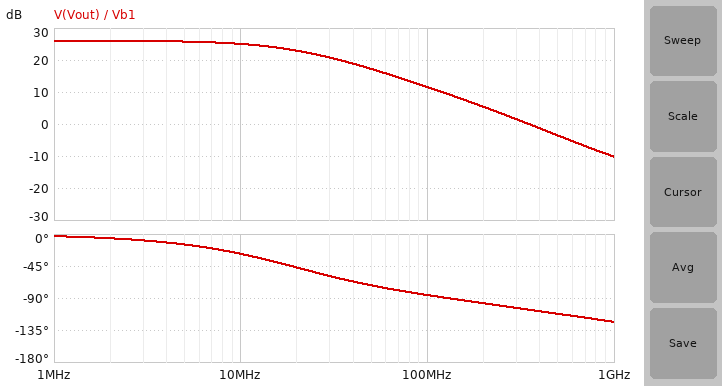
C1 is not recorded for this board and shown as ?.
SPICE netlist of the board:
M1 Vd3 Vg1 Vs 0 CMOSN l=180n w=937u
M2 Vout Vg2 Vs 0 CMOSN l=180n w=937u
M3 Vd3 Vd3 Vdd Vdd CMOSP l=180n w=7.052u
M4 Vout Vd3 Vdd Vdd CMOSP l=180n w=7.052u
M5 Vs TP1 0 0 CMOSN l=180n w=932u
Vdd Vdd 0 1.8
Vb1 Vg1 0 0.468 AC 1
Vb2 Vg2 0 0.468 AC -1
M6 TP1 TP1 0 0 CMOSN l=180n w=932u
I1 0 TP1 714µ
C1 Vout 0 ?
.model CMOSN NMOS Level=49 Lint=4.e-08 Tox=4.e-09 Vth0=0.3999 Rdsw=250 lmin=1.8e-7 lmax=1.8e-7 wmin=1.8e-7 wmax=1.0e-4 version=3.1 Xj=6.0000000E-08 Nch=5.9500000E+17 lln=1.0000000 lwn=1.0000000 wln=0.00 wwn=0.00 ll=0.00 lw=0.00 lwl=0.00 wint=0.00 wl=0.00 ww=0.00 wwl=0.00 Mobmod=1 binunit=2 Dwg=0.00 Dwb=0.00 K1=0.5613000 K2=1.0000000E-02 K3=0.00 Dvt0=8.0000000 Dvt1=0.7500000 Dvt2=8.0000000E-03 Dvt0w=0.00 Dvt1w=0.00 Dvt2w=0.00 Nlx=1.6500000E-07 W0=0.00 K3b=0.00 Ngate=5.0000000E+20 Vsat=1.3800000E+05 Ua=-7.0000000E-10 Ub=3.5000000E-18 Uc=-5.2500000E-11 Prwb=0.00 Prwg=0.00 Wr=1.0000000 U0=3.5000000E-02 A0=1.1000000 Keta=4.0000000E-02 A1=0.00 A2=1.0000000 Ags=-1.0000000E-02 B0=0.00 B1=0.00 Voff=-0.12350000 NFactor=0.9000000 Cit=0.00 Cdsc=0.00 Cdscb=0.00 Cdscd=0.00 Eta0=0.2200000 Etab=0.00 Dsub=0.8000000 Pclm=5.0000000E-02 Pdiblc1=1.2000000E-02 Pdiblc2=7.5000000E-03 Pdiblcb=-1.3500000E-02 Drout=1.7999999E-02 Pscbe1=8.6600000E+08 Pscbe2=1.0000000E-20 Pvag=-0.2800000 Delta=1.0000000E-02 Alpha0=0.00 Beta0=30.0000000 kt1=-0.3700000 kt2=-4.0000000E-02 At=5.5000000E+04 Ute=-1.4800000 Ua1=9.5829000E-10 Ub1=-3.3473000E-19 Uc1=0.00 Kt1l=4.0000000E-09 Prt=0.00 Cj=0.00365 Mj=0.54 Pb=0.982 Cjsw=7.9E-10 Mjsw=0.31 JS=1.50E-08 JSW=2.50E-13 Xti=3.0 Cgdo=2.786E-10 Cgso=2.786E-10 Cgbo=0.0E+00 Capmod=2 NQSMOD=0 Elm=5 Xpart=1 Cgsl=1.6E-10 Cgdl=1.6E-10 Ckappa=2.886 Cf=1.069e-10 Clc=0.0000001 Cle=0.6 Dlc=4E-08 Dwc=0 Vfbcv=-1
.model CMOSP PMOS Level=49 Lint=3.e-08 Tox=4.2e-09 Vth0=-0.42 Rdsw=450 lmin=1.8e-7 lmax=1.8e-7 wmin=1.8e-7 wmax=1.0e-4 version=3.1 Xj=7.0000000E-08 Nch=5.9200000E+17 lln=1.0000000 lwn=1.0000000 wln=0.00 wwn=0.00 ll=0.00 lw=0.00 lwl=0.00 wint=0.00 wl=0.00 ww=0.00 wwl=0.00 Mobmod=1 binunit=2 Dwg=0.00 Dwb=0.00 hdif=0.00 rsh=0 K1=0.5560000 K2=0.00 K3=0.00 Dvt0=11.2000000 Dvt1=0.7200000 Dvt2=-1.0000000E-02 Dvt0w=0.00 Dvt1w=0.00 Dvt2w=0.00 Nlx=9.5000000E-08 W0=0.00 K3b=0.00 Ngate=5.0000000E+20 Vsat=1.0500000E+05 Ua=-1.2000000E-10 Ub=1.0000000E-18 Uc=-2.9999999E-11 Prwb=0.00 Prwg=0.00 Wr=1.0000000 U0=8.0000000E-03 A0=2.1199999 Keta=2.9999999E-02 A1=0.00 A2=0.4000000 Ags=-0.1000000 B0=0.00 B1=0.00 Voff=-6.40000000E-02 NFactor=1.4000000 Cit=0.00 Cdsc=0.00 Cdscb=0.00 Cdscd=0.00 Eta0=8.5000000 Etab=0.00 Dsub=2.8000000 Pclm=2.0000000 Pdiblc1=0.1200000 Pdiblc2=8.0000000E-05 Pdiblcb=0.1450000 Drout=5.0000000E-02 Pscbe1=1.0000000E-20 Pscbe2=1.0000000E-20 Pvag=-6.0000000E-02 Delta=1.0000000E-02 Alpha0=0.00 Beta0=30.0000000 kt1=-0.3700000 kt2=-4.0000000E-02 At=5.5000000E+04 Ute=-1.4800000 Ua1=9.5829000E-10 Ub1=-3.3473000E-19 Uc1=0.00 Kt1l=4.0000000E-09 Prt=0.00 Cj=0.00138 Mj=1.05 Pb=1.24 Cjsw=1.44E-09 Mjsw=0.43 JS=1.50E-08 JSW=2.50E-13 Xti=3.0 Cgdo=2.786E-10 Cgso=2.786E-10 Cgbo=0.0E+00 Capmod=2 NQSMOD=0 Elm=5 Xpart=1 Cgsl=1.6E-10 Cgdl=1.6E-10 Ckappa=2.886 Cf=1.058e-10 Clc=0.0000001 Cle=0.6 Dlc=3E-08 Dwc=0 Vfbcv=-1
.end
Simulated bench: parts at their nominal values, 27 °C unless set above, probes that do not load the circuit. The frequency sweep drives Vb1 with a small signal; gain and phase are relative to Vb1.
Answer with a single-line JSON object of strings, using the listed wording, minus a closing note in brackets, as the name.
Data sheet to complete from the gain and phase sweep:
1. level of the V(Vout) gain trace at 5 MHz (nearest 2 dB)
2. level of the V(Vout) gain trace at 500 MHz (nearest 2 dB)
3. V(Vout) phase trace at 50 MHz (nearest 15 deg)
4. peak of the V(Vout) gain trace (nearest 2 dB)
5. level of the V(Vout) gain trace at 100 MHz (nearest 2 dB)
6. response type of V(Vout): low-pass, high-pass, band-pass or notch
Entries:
{"level of the V(Vout) gain trace at 5 MHz": "26 dB", "level of the V(Vout) gain trace at 500 MHz": "-4 dB", "V(Vout) phase trace at 50 MHz": "-75 deg", "peak of the V(Vout) gain trace": "26 dB", "level of the V(Vout) gain trace at 100 MHz": "12 dB", "response type of V(Vout): low-pass, high-pass, band-pass or notch": "low-pass"}
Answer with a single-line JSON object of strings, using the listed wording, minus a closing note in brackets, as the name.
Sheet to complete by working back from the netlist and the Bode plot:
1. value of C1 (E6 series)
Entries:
{"value of C1": "3.3 pF"}
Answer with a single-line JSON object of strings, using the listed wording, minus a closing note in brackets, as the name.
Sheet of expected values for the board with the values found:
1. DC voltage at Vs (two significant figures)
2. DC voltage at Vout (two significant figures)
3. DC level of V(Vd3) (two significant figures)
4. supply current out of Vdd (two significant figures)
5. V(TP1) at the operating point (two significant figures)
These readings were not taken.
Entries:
{"DC voltage at Vs": "190 mV", "DC voltage at Vout": "1.1 V", "DC level of V(Vd3)": "1.1 V", "supply current out of Vdd": "530 µA", "V(TP1) at the operating point": "340 mV"}
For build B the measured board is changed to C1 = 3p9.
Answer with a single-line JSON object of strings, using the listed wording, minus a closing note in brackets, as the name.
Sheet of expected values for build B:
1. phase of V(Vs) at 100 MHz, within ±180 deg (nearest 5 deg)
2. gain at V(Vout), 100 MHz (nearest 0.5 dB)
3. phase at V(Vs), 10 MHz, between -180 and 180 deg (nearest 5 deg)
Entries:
{"phase of V(Vs) at 100 MHz, within ±180 deg": "-155 deg", "gain at V(Vout), 100 MHz": "10.5 dB", "phase at V(Vs), 10 MHz, between -180 and 180 deg": "-40 deg"}
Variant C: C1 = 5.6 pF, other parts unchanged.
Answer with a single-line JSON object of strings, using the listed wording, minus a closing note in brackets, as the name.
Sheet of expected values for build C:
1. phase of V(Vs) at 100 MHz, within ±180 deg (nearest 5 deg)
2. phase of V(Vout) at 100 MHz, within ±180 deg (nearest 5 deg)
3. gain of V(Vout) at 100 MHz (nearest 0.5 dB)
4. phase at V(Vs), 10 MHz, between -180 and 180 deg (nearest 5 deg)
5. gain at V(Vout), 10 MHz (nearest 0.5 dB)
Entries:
{"phase of V(Vs) at 100 MHz, within ±180 deg": "-165 deg", "phase of V(Vout) at 100 MHz, within ±180 deg": "-90 deg", "gain of V(Vout) at 100 MHz": "8.0 dB", "phase at V(Vs), 10 MHz, between -180 and 180 deg": "-50 deg", "gain at V(Vout), 10 MHz": "24.0 dB"}
